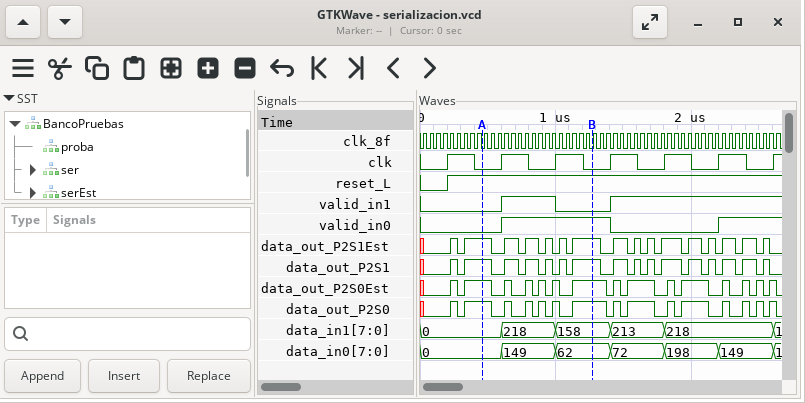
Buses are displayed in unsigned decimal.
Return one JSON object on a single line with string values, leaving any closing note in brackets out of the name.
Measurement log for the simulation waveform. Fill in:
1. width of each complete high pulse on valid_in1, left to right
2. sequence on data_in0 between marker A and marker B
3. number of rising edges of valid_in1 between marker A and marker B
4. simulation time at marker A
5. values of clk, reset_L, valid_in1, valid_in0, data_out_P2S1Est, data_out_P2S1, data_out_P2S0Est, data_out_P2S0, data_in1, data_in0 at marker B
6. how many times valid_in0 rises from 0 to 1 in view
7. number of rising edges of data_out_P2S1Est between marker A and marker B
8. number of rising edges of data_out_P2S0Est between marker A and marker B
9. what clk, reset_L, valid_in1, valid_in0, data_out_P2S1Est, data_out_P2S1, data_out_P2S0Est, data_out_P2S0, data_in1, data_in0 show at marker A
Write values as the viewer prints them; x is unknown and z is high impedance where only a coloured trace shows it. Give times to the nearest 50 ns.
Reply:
{"width of each complete high pulse on valid_in1, left to right": "400 ns", "sequence on data_in0 between marker A and marker B": "0, 149, 62", "number of rising edges of valid_in1 between marker A and marker B": "1", "simulation time at marker A": "450 ns", "values of clk, reset_L, valid_in1, valid_in0, data_out_P2S1Est, data_out_P2S1, data_out_P2S0Est, data_out_P2S0, data_in1, data_in0 at marker B": "clk=0, reset_L=1, valid_in1=0, valid_in0=1, data_out_P2S1Est=1, data_out_P2S1=1, data_out_P2S0Est=1, data_out_P2S0=1, data_in1=158, data_in0=62", "how many times valid_in0 rises from 0 to 1 in view": "2", "number of rising edges of data_out_P2S1Est between marker A and marker B": "5", "number of rising edges of data_out_P2S0Est between marker A and marker B": "5", "what clk, reset_L, valid_in1, valid_in0, data_out_P2S1Est, data_out_P2S1, data_out_P2S0Est, data_out_P2S0, data_in1, data_in0 show at marker A": "clk=0, reset_L=1, valid_in1=0, valid_in0=0, data_out_P2S1Est=1, data_out_P2S1=1, data_out_P2S0Est=1, data_out_P2S0=1, data_in1=0, data_in0=0"}
